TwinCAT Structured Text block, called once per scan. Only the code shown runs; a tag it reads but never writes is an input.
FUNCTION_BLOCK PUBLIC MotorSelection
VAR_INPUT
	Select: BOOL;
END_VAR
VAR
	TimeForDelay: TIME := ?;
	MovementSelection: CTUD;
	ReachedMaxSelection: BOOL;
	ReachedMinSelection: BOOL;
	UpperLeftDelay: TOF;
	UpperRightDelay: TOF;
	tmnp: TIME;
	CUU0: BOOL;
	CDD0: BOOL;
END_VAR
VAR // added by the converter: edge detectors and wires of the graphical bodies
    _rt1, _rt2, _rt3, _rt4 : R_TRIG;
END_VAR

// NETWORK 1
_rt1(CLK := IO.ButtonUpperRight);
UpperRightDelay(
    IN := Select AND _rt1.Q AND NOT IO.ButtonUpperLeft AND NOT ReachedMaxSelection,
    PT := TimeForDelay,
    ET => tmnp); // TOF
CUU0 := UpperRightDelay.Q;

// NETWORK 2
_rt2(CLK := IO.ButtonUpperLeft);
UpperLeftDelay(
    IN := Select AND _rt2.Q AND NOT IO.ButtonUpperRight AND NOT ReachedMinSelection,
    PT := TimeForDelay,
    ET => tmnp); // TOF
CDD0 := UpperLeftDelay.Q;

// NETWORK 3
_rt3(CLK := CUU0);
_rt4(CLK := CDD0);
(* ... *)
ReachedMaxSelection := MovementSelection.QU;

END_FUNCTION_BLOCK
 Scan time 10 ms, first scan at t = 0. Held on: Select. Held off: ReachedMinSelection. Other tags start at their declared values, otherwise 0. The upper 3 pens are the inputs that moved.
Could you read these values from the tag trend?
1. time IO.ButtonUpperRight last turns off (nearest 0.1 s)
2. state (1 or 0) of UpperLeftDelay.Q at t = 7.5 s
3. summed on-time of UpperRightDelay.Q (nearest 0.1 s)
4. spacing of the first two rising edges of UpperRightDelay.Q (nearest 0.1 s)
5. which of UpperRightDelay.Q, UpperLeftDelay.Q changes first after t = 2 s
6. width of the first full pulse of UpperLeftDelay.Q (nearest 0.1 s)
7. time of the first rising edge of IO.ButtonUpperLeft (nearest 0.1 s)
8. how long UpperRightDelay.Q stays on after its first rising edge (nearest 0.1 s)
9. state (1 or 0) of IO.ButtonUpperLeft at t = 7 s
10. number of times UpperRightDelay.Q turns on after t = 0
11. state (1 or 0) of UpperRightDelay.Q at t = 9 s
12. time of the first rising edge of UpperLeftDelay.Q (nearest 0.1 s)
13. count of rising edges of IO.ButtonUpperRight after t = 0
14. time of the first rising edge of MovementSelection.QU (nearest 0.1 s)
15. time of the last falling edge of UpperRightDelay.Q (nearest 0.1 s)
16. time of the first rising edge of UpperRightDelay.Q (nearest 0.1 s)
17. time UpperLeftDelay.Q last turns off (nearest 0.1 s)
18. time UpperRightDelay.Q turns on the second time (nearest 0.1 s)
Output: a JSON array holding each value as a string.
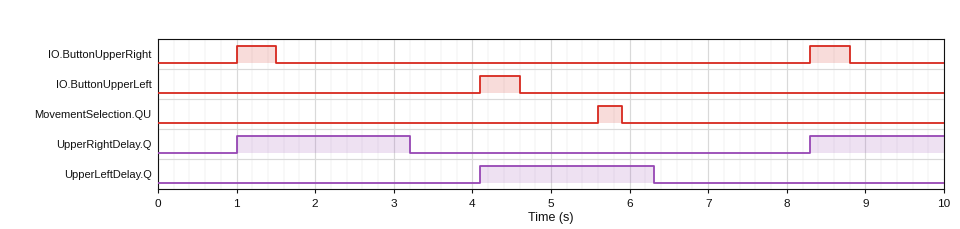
["8.8 s", "0", "3.9 s", "7.3 s", "UpperRightDelay.Q", "2.2 s", "4.1 s", "2.2 s", "0", "2", "1", "4.1 s", "2", "5.6 s", "3.2 s", "1.0 s", "6.3 s", "8.3 s"]
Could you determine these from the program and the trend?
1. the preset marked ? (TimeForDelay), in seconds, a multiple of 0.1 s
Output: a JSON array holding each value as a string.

["2.2 s"]
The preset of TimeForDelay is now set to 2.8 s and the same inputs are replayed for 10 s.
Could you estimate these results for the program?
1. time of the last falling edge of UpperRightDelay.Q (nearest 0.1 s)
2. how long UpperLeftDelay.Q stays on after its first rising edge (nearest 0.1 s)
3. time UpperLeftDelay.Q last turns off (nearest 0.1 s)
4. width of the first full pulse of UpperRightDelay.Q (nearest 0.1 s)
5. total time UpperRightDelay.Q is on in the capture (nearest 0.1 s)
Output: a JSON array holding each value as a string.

["3.8 s", "2.8 s", "6.9 s", "2.8 s", "4.5 s"]
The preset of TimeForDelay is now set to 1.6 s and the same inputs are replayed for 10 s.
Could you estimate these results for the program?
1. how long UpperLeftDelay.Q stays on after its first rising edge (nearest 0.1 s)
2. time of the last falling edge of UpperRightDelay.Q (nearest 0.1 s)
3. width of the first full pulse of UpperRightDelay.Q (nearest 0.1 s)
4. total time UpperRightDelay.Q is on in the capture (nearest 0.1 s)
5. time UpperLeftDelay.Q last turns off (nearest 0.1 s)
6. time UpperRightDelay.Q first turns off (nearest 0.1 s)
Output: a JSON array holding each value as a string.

["1.6 s", "9.9 s", "1.6 s", "3.2 s", "5.7 s", "2.6 s"]
